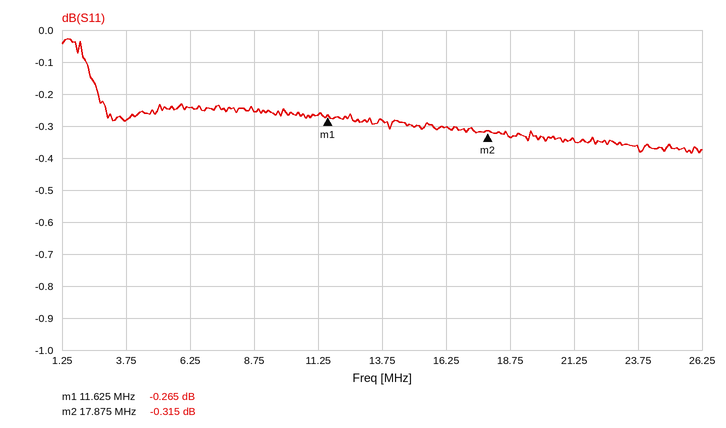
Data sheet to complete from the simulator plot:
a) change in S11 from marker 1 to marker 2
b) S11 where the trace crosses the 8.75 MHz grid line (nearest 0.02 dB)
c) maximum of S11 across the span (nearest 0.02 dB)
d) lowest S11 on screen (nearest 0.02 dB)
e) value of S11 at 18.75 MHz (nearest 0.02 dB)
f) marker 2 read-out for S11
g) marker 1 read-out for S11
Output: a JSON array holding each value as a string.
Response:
["-0.050 dB", "-0.26 dB", "-0.02 dB", "-0.38 dB", "-0.34 dB", "-0.315 dB", "-0.265 dB"]
